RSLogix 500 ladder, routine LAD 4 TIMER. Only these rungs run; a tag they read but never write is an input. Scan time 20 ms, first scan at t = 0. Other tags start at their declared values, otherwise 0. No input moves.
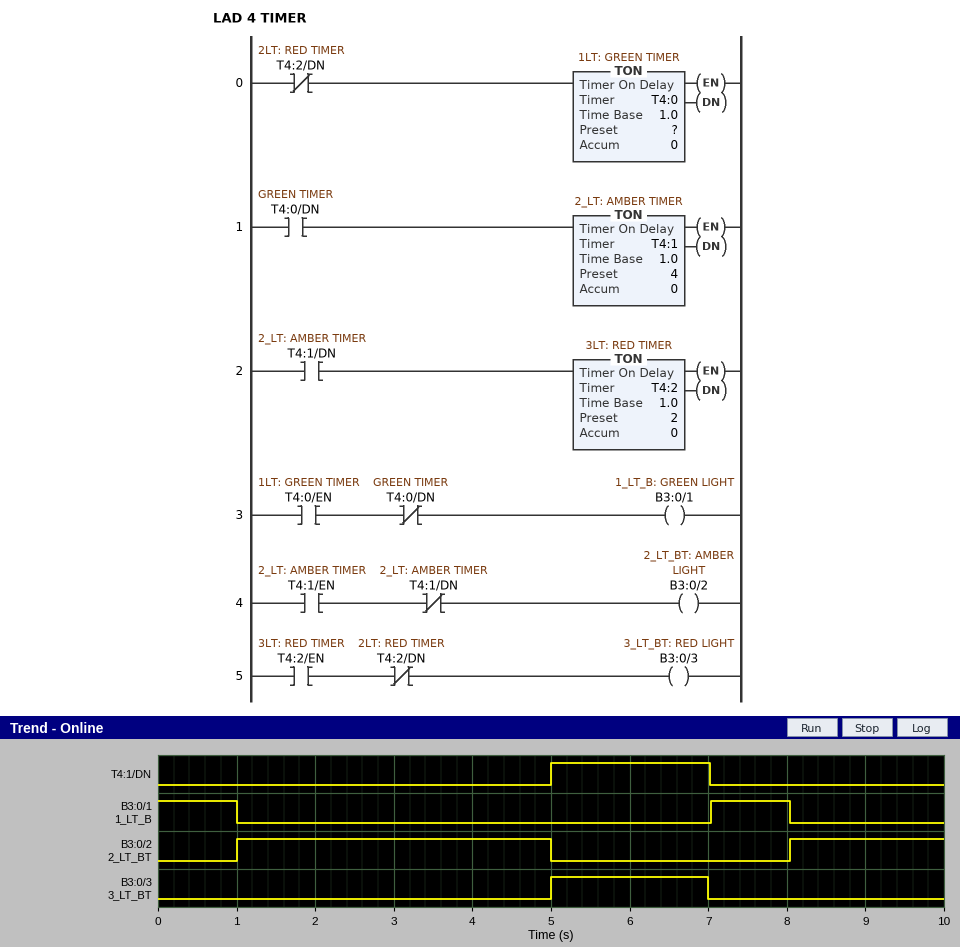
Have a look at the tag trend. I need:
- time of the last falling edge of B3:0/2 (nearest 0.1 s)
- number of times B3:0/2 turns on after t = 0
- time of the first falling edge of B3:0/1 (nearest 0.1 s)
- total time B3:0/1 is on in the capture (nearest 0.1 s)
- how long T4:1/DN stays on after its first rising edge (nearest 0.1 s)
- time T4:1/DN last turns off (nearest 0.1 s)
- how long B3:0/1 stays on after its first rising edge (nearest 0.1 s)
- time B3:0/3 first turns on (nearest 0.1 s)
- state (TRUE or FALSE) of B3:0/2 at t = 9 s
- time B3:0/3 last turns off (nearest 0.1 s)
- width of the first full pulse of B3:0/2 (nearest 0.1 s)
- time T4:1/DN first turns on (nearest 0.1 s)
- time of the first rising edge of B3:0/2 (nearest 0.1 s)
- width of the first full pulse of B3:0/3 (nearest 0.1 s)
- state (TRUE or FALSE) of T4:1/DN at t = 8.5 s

5.0 s
2
1.0 s
2.0 s
2.0 s
7.0 s
1.0 s
5.0 s
TRUE
7.0 s
4.0 s
5.0 s
1.0 s
2.0 s
FALSE
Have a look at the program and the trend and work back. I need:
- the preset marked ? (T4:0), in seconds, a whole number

1 s
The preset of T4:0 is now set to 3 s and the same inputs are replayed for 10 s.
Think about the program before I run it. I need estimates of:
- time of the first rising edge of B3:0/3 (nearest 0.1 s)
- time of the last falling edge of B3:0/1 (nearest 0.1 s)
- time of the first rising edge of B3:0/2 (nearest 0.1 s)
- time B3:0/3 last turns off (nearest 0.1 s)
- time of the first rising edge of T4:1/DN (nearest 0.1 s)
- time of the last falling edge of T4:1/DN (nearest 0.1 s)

7.0 s
3.0 s
3.0 s
9.0 s
7.0 s
9.0 s
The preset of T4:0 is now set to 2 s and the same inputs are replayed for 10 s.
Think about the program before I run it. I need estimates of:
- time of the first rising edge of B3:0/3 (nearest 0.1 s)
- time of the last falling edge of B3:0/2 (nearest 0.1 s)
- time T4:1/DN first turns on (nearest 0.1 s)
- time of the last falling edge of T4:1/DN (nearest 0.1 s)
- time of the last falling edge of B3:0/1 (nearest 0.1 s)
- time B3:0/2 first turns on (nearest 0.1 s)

6.0 s
6.0 s
6.0 s
8.0 s
2.0 s
2.0 s
